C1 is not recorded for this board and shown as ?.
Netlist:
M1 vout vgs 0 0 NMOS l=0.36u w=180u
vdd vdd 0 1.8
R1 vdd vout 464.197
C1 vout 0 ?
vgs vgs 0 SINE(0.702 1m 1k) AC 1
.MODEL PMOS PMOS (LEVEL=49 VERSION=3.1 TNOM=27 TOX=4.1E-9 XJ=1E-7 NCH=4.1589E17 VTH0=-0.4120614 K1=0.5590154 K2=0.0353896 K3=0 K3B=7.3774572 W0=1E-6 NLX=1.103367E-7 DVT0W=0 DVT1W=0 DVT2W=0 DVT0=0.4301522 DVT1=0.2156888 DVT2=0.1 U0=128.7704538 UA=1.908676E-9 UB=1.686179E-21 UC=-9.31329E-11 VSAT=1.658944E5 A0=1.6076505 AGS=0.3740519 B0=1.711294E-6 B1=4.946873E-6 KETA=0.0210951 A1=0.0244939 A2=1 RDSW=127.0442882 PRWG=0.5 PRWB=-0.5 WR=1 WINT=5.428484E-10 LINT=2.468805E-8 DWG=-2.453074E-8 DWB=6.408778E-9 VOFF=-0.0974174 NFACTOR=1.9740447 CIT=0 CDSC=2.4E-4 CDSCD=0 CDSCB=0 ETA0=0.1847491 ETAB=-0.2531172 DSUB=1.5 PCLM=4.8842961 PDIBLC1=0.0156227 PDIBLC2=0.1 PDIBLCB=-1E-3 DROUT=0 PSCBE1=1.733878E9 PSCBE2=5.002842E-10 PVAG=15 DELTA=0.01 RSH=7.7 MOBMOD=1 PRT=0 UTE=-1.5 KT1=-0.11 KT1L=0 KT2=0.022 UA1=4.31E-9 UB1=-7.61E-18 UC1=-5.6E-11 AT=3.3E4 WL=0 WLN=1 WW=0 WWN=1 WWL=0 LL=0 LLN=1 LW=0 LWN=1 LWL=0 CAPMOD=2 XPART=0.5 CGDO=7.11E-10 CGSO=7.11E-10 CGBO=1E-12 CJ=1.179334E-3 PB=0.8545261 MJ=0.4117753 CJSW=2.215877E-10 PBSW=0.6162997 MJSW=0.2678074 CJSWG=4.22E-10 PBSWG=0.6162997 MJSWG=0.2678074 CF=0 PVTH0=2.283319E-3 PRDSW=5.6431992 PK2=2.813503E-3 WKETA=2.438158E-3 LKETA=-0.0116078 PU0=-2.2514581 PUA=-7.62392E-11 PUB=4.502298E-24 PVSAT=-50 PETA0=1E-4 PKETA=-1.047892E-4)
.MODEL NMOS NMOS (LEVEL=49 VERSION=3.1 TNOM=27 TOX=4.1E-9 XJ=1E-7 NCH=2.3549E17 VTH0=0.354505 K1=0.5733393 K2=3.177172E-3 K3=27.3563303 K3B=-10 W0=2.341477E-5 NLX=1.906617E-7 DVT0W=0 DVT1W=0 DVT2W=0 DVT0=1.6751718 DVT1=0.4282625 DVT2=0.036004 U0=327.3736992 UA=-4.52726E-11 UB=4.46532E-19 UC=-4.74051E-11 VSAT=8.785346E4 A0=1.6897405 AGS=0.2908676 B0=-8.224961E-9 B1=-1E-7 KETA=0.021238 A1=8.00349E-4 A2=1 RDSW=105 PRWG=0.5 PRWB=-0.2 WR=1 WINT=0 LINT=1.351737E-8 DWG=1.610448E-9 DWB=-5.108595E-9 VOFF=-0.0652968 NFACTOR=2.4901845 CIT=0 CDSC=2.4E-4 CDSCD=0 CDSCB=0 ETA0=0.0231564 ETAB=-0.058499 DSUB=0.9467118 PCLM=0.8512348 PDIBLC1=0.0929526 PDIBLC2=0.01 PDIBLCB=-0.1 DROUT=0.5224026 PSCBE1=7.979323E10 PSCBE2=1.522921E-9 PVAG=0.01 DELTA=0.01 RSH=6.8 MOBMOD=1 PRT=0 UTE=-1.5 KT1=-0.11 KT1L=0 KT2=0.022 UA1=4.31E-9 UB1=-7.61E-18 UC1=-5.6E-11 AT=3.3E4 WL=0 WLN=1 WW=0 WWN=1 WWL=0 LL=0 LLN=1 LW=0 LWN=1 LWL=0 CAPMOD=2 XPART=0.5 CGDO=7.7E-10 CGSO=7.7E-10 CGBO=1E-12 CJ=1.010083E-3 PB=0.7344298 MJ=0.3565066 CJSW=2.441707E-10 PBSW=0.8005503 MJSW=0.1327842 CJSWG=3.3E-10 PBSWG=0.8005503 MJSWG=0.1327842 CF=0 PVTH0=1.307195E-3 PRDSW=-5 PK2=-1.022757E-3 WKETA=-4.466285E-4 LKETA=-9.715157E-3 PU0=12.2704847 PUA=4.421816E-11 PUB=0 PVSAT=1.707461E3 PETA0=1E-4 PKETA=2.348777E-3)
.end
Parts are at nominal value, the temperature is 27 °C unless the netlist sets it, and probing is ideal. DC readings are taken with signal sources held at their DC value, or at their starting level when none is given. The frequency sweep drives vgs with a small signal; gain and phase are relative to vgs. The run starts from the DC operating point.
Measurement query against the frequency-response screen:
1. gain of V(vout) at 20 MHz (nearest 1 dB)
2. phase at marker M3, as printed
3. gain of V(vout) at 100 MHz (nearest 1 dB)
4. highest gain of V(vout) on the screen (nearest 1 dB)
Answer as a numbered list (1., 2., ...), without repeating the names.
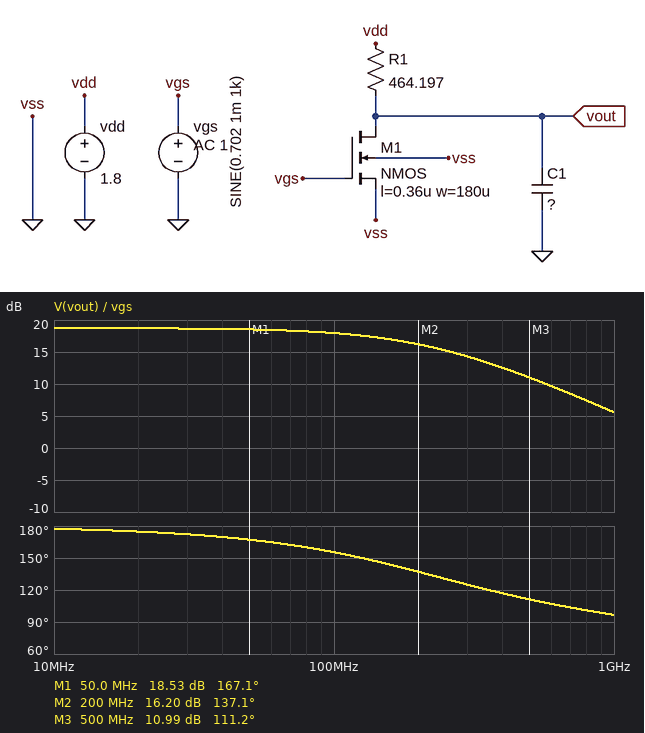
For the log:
1. 19 dB
2. 111.2 deg
3. 18 dB
4. 19 dB
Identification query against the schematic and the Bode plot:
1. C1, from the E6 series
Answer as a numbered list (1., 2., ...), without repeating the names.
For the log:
1. 1.5 pF
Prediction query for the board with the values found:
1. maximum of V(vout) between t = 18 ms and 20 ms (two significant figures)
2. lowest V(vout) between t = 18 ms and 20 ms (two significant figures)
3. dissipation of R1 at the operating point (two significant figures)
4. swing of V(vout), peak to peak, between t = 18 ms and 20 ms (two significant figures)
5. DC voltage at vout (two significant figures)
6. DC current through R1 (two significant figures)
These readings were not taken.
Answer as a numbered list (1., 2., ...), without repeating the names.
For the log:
1. 660 mV
2. 640 mV
3. 2.9 mW
4. 17 mV
5. 650 mV
6. 2.5 mA
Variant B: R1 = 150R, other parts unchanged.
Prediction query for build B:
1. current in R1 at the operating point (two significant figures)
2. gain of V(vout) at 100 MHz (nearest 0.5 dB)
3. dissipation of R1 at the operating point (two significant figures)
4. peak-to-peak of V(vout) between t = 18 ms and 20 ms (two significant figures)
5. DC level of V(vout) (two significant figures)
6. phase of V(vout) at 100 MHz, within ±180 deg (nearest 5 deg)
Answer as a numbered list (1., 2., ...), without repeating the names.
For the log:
1. 2.6 mA
2. 10.0 dB
3. 1.0 mW
4. 6.3 mV
5. 1.4 V
6. 170 deg
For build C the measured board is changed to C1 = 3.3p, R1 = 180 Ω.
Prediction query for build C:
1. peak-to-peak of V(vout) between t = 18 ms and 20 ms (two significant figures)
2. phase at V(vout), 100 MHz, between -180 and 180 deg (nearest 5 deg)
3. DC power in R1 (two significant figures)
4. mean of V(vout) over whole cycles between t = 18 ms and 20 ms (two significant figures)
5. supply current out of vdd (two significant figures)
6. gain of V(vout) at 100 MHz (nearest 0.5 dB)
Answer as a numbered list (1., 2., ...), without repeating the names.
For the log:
1. 7.4 mV
2. 160 deg
3. 1.2 mW
4. 1.3 V
5. 2.6 mA
6. 11.0 dB
